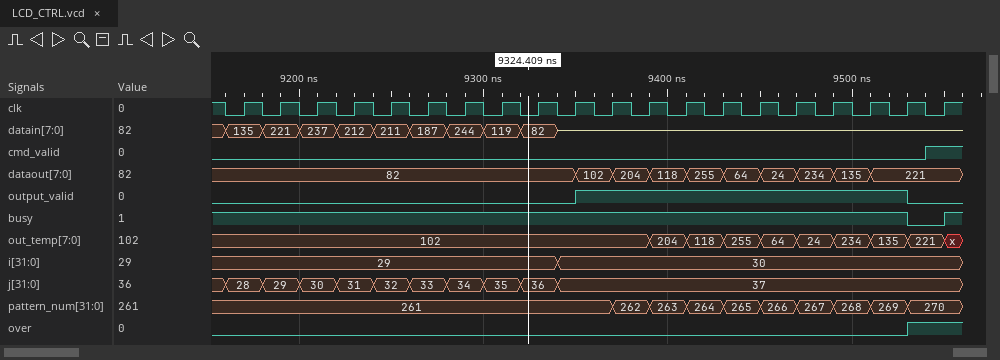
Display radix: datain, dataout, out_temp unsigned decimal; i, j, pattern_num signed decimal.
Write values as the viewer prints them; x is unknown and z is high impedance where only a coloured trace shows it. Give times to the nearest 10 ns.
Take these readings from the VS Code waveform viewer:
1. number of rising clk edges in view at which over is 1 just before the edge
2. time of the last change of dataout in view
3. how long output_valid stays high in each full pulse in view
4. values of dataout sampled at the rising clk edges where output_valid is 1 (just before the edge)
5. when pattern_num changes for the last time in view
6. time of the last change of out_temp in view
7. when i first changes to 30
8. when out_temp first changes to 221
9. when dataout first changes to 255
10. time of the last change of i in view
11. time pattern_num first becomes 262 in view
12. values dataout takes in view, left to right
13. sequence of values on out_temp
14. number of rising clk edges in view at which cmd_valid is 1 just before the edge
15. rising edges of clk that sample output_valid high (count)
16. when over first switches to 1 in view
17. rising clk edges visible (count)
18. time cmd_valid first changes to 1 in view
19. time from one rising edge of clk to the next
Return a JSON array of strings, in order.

["1", "9510 ns", "180 ns", "102, 204, 118, 255, 64, 24, 234, 135, 221", "9530 ns", "9550 ns", "9340 ns", "9530 ns", "9410 ns", "9340 ns", "9370 ns", "82, 102, 204, 118, 255, 64, 24, 234, 135, 221", "102, 204, 118, 255, 64, 24, 234, 135, 221, x", "1", "9", "9530 ns", "20", "9540 ns", "20 ns"]
